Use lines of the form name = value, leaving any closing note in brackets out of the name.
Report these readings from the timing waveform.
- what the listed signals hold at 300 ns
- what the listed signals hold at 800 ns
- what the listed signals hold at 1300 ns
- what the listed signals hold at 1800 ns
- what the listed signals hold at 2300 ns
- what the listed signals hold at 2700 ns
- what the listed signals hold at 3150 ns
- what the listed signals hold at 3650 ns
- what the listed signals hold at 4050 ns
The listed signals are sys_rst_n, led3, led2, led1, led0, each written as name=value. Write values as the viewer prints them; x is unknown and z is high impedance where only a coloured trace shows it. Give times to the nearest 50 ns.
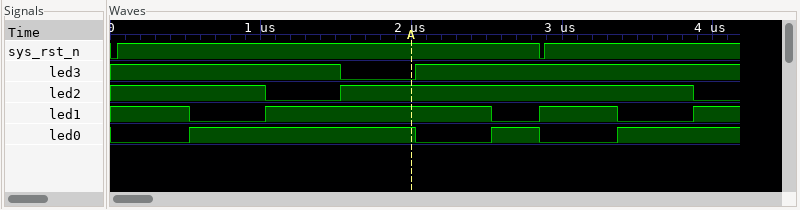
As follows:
what the listed signals hold at 300 ns = sys_rst_n=1, led3=1, led2=1, led1=1, led0=0
what the listed signals hold at 800 ns = sys_rst_n=1, led3=1, led2=1, led1=0, led0=1
what the listed signals hold at 1300 ns = sys_rst_n=1, led3=1, led2=0, led1=1, led0=1
what the listed signals hold at 1800 ns = sys_rst_n=1, led3=0, led2=1, led1=1, led0=1
what the listed signals hold at 2300 ns = sys_rst_n=1, led3=1, led2=1, led1=1, led0=0
what the listed signals hold at 2700 ns = sys_rst_n=1, led3=1, led2=1, led1=0, led0=1
what the listed signals hold at 3150 ns = sys_rst_n=1, led3=1, led2=1, led1=1, led0=0
what the listed signals hold at 3650 ns = sys_rst_n=1, led3=1, led2=1, led1=0, led0=1
what the listed signals hold at 4050 ns = sys_rst_n=1, led3=1, led2=0, led1=1, led0=1
